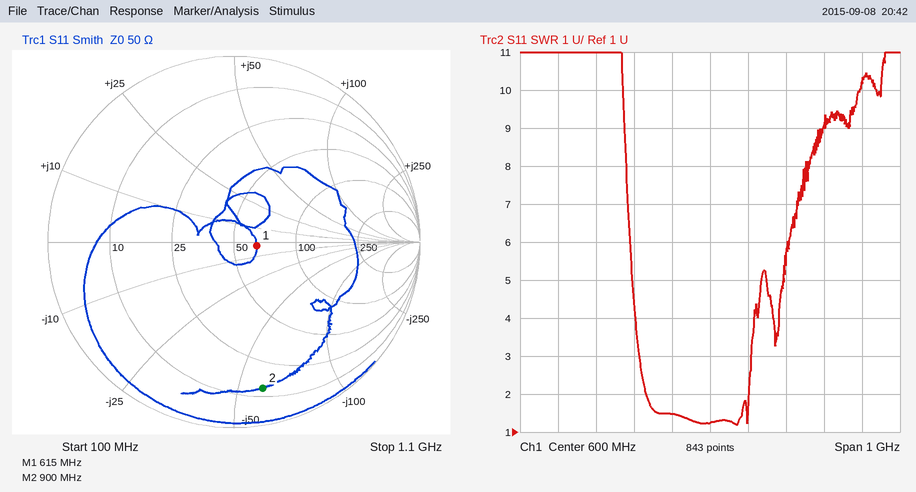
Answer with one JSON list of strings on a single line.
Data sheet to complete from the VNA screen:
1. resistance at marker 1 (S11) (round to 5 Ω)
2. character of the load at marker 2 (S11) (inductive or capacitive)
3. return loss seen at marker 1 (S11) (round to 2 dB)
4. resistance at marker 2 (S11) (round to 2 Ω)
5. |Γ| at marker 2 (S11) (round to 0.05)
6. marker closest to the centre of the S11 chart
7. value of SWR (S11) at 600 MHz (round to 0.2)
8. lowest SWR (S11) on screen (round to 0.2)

["65 Ω", "capacitive", "18 dB", "14 Ω", "0.80", "marker 1", "1.2", "1.2"]
